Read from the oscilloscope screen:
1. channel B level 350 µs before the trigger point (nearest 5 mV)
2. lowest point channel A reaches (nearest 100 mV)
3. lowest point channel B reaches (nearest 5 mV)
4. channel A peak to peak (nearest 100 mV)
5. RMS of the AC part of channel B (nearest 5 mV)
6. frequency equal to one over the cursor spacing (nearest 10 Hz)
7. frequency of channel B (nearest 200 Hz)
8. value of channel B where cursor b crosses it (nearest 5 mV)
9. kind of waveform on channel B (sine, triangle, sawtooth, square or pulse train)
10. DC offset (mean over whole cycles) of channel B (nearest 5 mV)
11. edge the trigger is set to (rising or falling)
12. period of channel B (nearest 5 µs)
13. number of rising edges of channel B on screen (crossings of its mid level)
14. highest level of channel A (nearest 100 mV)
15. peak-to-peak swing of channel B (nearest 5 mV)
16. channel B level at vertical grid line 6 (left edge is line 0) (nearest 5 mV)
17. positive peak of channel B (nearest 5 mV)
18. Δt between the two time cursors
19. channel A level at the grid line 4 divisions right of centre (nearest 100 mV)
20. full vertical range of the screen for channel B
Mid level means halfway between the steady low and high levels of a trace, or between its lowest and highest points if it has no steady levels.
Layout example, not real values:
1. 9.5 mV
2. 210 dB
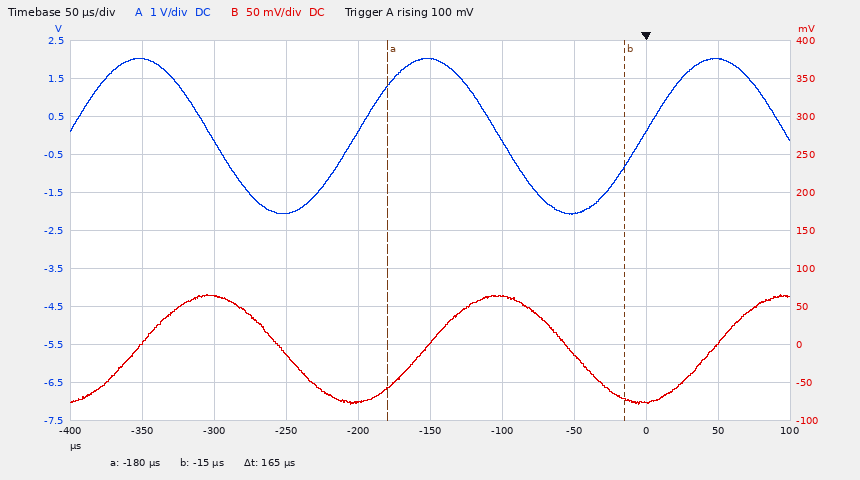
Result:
1. 0 mV
2. -2.1 V
3. -80 mV
4. 4.1 V
5. 50 mV
6. 6.06 kHz
7. 5.0 kHz
8. -70 mV
9. sine
10. -5 mV
11. rising
12. 200 µs
13. 3
14. 2.0 V
15. 145 mV
16. 65 mV
17. 65 mV
18. 165 µs
19. 2.0 V
20. 500 mV
